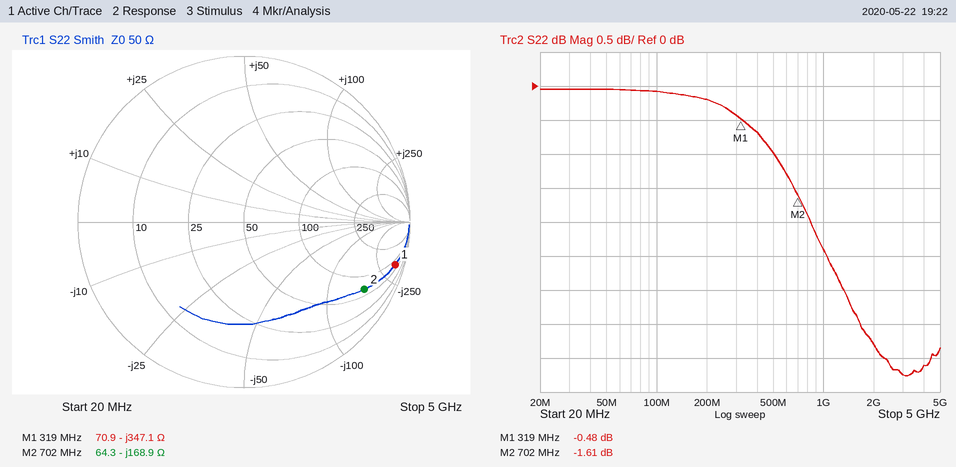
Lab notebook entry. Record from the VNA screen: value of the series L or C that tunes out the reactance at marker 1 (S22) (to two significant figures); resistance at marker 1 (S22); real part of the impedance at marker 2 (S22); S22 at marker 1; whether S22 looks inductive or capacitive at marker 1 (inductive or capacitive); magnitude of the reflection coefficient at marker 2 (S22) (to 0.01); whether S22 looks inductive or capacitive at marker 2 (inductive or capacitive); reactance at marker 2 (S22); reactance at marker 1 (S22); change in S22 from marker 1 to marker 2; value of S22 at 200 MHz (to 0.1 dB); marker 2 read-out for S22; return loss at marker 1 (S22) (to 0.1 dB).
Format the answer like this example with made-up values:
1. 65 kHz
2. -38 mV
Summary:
1. 170 nH
2. 70.9 Ω
3. 64.3 Ω
4. -0.48 dB
5. capacitive
6. 0.83
7. capacitive
8. -168.9 Ω
9. -347.1 Ω
10. -1.13 dB
11. -0.2 dB
12. -1.61 dB
13. 0.5 dB
